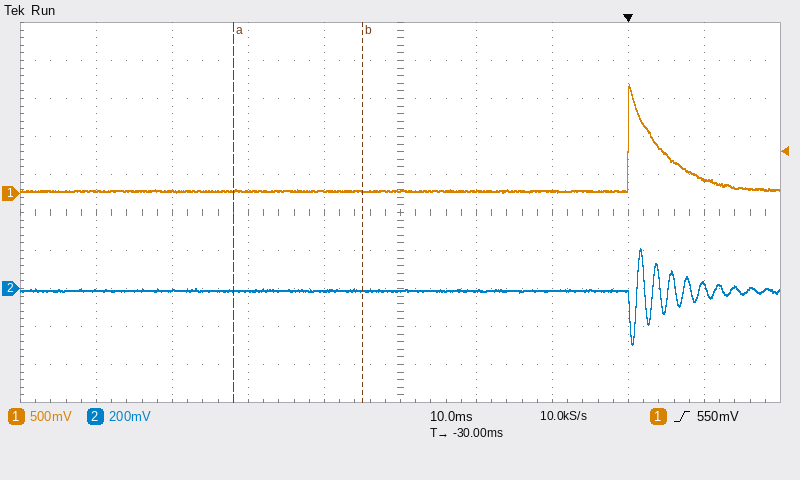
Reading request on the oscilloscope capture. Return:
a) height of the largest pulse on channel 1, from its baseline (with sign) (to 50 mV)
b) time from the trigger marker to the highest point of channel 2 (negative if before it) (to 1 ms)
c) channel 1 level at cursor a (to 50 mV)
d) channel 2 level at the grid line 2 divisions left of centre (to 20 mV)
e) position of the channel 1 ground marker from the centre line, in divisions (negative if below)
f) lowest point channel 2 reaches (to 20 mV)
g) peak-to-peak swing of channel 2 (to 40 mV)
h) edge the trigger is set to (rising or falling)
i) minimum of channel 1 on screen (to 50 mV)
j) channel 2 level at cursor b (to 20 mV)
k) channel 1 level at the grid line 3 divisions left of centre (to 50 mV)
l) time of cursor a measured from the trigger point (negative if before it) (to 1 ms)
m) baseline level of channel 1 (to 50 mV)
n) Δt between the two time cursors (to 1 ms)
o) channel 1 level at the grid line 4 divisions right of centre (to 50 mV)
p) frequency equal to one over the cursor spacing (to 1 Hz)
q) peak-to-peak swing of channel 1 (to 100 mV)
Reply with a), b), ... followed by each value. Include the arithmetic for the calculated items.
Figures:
a) +1.40 V
b) +2 ms
c) 50 mV
d) -20 mV
e) +0.5 div
f) -300 mV
g) 520 mV
h) rising
i) 0 mV
j) -20 mV
k) 50 mV
l) -52 ms
m) 50 mV
n) 17 ms
o) 200 mV
p) 1 / 17 ms ≈ 59 Hz
q) 1.40 V
